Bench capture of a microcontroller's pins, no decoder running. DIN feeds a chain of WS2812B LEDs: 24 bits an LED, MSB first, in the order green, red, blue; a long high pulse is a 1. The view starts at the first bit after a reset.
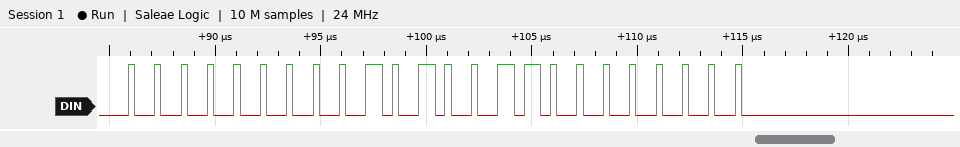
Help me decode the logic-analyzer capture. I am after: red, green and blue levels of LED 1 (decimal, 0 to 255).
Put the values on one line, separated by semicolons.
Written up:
83, 0, 0
